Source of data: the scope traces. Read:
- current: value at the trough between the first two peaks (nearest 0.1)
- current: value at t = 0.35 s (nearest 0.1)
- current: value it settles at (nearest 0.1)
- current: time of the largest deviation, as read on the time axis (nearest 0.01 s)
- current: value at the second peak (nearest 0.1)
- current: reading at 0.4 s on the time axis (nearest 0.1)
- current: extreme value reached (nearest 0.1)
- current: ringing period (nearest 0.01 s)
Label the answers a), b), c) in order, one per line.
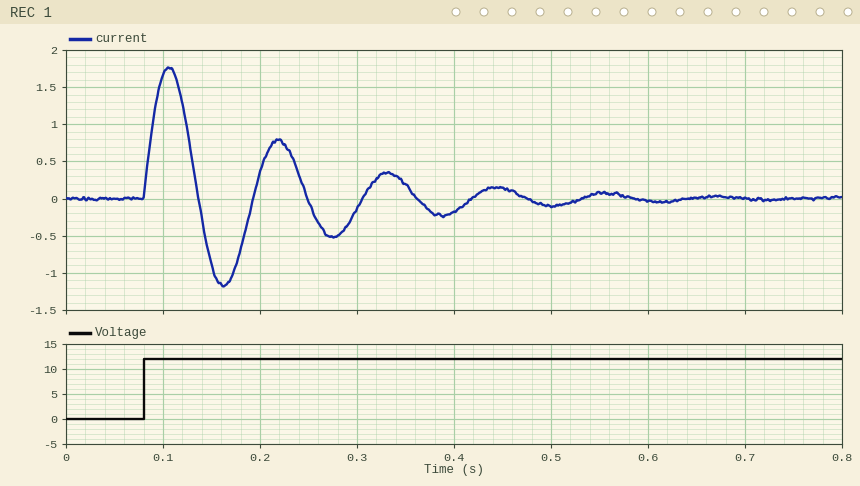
a) -1.2
b) 0.2
c) 0.0
d) 0.11 s
e) 0.8
f) -0.2
g) 1.8
h) 0.11 s
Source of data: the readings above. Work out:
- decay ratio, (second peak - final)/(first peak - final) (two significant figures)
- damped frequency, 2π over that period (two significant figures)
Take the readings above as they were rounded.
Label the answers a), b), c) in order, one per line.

a) 0.44
b) 57 rad/s
